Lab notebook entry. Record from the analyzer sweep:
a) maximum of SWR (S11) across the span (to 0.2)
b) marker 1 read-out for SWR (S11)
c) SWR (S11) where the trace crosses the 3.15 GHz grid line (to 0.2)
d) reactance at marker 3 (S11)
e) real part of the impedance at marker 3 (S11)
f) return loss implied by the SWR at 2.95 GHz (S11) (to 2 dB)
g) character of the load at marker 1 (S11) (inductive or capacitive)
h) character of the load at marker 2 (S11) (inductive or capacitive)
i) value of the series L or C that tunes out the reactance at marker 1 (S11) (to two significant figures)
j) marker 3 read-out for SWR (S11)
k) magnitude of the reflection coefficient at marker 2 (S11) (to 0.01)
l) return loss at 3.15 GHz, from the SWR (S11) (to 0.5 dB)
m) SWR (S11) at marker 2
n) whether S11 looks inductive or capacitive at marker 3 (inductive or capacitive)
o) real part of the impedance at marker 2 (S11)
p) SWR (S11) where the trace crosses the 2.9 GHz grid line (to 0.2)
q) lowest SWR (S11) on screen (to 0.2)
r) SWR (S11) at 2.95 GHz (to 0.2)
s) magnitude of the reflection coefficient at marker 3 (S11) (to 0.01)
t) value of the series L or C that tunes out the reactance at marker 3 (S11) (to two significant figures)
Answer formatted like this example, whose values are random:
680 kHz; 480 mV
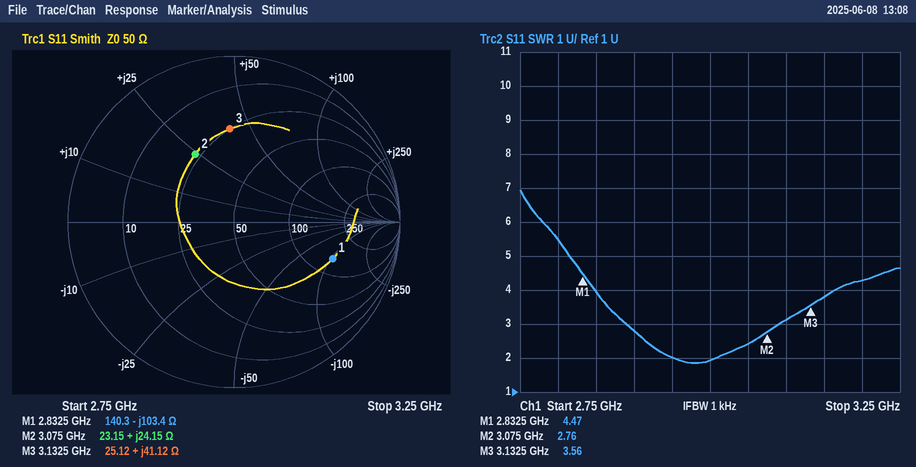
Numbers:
7.0; 4.47; 3.8; +41.12 Ω; 25.12 Ω; 10 dB; capacitive; inductive; 5.8 nH; 3.56; 0.47; 4.5 dB; 2.76; inductive; 23.15 Ω; 2.8; 1.8; 2.0; 0.56; 1.2 pF
